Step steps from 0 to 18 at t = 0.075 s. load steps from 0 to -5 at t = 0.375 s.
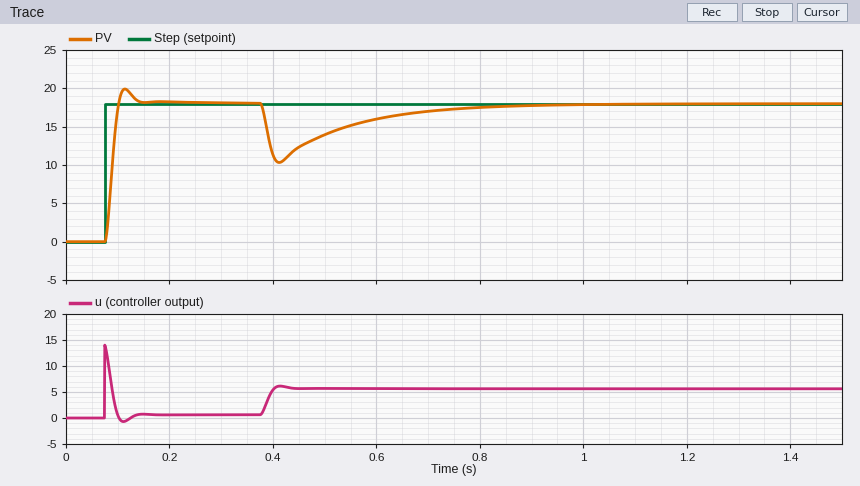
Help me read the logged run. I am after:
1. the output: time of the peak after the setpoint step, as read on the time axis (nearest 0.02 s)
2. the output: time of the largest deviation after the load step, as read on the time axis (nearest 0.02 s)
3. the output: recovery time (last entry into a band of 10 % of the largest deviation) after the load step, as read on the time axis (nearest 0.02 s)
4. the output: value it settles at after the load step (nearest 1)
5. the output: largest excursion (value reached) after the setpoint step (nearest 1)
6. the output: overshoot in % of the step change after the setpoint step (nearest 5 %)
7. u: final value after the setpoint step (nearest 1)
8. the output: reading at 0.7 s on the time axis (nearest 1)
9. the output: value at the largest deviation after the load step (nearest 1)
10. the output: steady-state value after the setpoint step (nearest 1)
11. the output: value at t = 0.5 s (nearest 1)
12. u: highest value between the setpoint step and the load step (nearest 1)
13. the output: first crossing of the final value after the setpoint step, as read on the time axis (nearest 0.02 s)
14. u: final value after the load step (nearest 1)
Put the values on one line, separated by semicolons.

0.12 s; 0.42 s; 0.74 s; 18; 20; 10 %; 1; 17; 10; 18; 14; 14; 0.10 s; 6
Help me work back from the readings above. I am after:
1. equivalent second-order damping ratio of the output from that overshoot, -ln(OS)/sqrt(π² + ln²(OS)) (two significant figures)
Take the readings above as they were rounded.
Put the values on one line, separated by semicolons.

0.59
